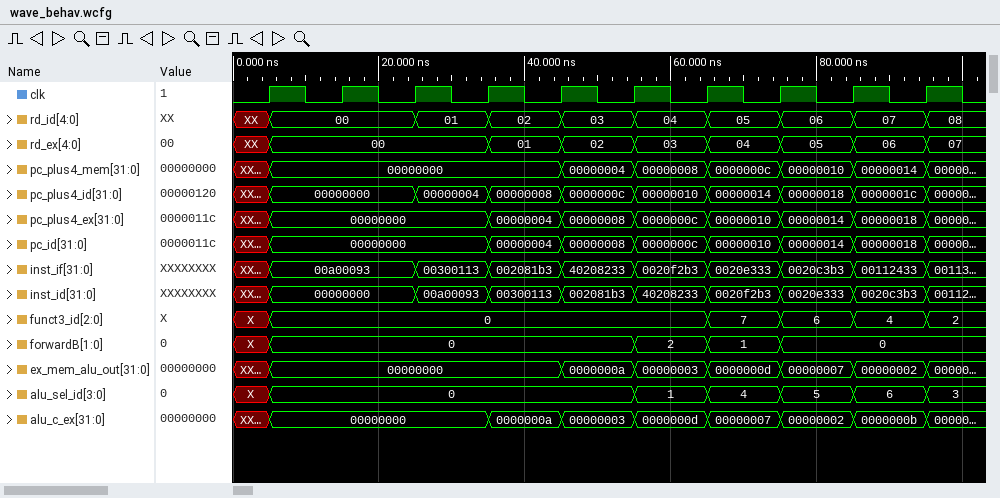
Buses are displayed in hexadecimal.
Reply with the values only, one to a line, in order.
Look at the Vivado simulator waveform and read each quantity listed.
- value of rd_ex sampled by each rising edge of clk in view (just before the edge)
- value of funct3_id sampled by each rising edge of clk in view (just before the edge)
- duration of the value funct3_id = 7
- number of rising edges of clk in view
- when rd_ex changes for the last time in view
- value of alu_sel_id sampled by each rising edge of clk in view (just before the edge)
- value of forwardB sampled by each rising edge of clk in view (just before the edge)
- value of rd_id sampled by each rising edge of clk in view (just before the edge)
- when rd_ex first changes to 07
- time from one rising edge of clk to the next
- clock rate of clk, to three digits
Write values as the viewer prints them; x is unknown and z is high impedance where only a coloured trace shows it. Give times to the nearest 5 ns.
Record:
XX, 00, 00, 00, 01, 02, 03, 04, 05, 06
X, 0, 0, 0, 0, 0, 0, 7, 6, 4
10 ns
10
95 ns
X, 0, 0, 0, 0, 0, 1, 4, 5, 6
X, 0, 0, 0, 0, 0, 2, 1, 0, 0
XX, 00, 00, 01, 02, 03, 04, 05, 06, 07
95 ns
10 ns
100 MHz
